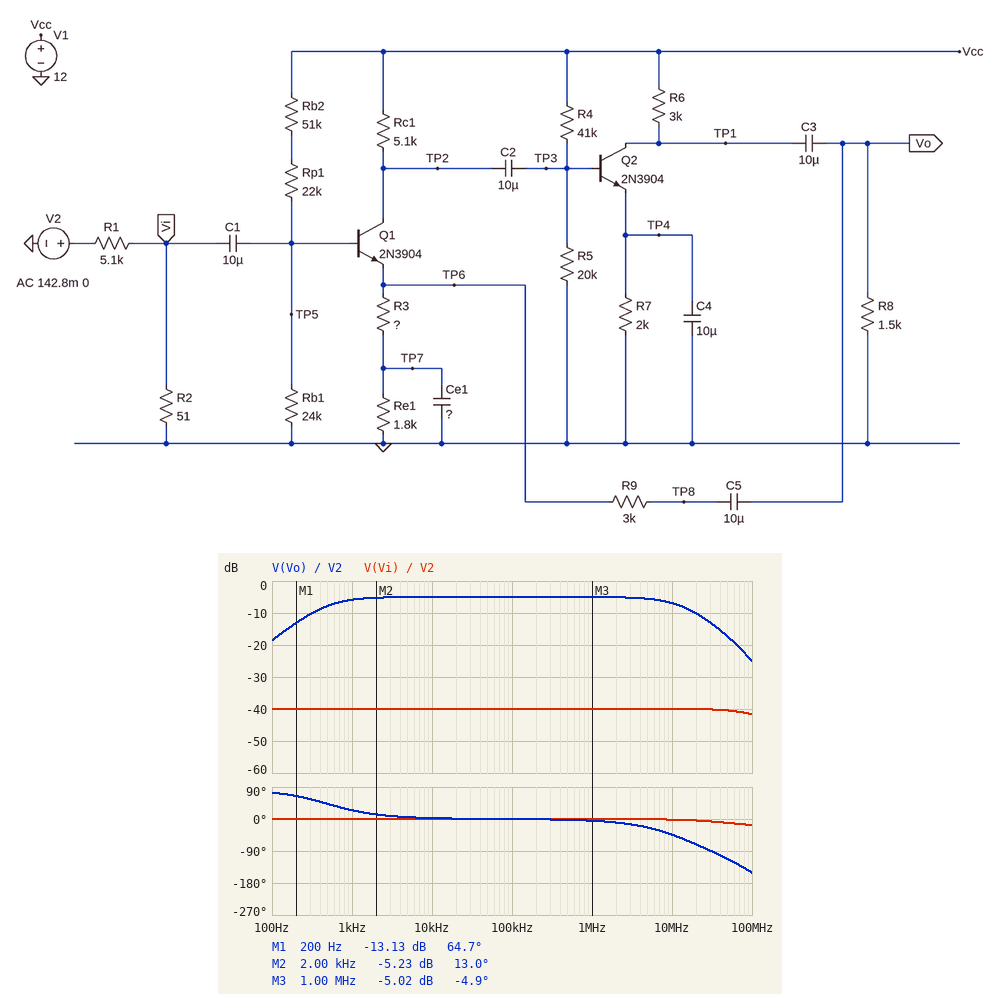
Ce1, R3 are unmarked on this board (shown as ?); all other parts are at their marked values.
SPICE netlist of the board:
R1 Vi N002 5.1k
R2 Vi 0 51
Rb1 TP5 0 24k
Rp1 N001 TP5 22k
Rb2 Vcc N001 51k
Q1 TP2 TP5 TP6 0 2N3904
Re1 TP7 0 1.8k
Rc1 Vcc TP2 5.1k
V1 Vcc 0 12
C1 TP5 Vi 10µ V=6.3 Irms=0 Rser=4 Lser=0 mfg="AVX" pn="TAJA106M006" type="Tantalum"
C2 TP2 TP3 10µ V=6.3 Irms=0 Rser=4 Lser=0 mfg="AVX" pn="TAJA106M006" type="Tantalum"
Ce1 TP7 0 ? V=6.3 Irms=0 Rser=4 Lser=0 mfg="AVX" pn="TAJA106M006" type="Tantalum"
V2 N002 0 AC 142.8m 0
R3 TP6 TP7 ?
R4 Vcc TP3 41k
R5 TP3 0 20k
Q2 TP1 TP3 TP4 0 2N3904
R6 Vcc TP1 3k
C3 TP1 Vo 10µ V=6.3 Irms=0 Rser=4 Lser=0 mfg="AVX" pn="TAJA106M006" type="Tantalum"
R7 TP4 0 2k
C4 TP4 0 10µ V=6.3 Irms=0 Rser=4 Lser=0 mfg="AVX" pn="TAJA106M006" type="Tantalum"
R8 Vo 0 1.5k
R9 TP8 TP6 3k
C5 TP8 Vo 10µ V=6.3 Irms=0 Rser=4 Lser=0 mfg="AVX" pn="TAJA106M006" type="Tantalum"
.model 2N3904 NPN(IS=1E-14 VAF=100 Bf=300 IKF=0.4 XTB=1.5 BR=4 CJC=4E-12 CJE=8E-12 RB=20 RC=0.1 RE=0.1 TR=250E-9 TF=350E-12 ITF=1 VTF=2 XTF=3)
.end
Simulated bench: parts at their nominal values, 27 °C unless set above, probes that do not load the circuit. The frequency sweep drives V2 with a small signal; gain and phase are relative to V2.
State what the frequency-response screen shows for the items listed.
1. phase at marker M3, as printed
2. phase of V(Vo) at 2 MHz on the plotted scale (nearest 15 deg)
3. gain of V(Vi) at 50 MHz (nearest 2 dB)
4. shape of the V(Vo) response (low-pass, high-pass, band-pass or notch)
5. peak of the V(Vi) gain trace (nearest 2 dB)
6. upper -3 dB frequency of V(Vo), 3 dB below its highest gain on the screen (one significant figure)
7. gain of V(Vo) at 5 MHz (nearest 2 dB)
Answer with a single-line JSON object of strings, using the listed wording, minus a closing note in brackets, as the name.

{"phase at marker M3, as printed": "-4.9 deg", "phase of V(Vo) at 2 MHz on the plotted scale": "-15 deg", "gain of V(Vi) at 50 MHz": "-40 dB", "shape of the V(Vo) response": "band-pass", "peak of the V(Vi) gain trace": "-40 dB", "upper -3 dB frequency of V(Vo), 3 dB below its highest gain on the screen": "10 MHz", "gain of V(Vo) at 5 MHz": "-6 dB"}
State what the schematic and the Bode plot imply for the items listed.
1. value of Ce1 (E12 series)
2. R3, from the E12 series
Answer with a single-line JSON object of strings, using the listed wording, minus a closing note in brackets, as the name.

{"value of Ce1": "6.8 µF", "R3, from the E12 series": "47 Ω"}
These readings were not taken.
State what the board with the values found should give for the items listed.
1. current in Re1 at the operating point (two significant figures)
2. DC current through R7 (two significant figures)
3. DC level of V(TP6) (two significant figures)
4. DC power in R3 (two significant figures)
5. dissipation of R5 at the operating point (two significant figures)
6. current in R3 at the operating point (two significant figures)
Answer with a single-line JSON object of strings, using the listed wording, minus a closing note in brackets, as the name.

{"current in Re1 at the operating point": "1.2 mA", "DC current through R7": "1.6 mA", "DC level of V(TP6)": "2.2 V", "DC power in R3": "69 µW", "dissipation of R5 at the operating point": "750 µW", "current in R3 at the operating point": "1.2 mA"}
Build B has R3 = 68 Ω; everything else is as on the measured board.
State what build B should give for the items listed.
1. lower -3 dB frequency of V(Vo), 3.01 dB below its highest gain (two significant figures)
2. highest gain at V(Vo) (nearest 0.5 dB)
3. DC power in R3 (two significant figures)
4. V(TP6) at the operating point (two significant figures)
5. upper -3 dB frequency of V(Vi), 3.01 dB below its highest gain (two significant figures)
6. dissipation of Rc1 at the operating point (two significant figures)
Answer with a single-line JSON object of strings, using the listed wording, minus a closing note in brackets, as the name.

{"lower -3 dB frequency of V(Vo), 3.01 dB below its highest gain": "340 Hz", "highest gain at V(Vo)": "-8.0 dB", "DC power in R3": "98 µW", "V(TP6) at the operating point": "2.2 V", "upper -3 dB frequency of V(Vi), 3.01 dB below its highest gain": "220 MHz", "dissipation of Rc1 at the operating point": "7.3 mW"}
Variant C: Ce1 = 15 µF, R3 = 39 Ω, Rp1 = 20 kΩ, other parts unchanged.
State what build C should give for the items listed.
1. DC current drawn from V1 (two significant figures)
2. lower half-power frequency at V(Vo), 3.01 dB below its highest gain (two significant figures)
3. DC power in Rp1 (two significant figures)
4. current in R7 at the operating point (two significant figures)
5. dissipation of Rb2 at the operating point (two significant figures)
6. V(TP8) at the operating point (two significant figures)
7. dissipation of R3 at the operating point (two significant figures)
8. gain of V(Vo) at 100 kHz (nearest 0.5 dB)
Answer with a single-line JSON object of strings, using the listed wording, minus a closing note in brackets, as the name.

{"DC current drawn from V1": "3.2 mA", "lower half-power frequency at V(Vo), 3.01 dB below its highest gain": "260 Hz", "DC power in Rp1": "320 µW", "current in R7 at the operating point": "1.6 mA", "dissipation of Rb2 at the operating point": "830 µW", "V(TP8) at the operating point": "2.3 V", "dissipation of R3 at the operating point": "61 µW", "gain of V(Vo) at 100 kHz": "-3.5 dB"}
